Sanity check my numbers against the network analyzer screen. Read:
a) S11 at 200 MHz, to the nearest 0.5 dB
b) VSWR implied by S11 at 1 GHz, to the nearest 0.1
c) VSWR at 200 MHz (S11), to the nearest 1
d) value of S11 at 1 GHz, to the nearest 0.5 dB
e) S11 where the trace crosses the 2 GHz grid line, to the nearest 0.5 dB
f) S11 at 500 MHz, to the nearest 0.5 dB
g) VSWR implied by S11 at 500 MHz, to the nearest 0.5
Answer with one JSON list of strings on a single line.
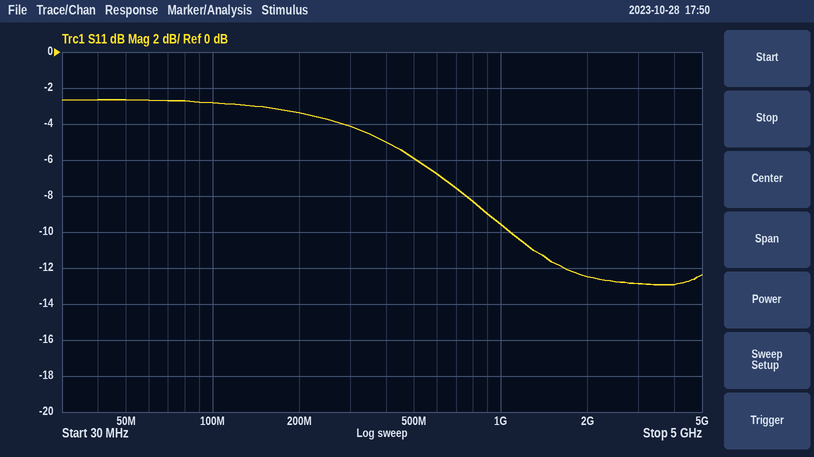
["-3.5 dB", "2.0", "5", "-9.5 dB", "-12.5 dB", "-6.0 dB", "3.0"]
